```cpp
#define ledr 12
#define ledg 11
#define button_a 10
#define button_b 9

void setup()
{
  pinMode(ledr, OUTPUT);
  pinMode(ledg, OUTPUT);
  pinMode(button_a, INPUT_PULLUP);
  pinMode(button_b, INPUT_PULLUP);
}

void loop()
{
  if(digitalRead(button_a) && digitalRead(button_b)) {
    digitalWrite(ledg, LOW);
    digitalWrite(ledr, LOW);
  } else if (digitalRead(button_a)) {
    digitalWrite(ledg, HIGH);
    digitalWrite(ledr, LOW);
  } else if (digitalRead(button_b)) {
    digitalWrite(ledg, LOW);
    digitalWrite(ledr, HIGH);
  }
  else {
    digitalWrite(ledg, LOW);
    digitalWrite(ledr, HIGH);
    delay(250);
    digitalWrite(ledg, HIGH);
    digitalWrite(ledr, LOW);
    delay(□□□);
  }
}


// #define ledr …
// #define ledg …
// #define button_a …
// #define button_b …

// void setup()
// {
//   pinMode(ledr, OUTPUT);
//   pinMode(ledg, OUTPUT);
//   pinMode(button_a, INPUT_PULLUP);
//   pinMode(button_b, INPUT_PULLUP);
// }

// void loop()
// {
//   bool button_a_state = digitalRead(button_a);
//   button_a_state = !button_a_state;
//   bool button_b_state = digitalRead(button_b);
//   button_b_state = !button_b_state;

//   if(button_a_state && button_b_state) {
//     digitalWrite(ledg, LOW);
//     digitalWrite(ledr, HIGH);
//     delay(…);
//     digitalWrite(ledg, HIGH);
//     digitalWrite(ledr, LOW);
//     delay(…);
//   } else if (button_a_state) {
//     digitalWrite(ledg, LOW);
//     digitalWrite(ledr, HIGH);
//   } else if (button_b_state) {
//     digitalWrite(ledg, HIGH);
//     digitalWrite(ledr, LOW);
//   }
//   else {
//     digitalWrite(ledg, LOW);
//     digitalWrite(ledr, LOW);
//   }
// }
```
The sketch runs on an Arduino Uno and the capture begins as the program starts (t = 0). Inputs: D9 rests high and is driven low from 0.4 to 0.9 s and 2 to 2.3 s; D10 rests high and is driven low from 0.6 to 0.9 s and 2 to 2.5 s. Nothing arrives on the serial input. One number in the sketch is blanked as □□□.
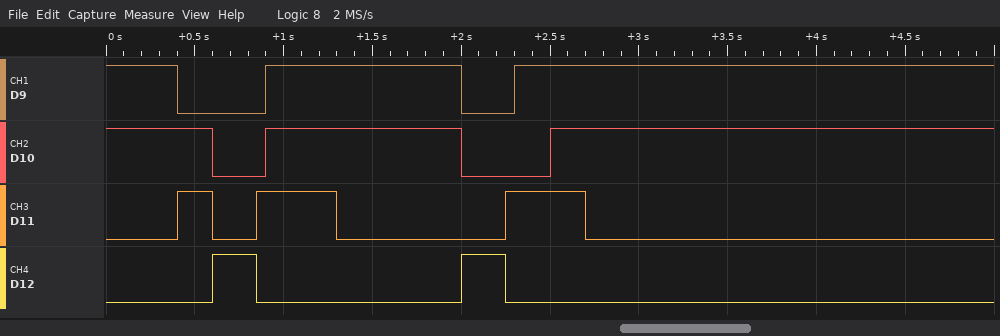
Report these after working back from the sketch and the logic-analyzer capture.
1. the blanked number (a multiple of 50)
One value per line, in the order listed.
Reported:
450
